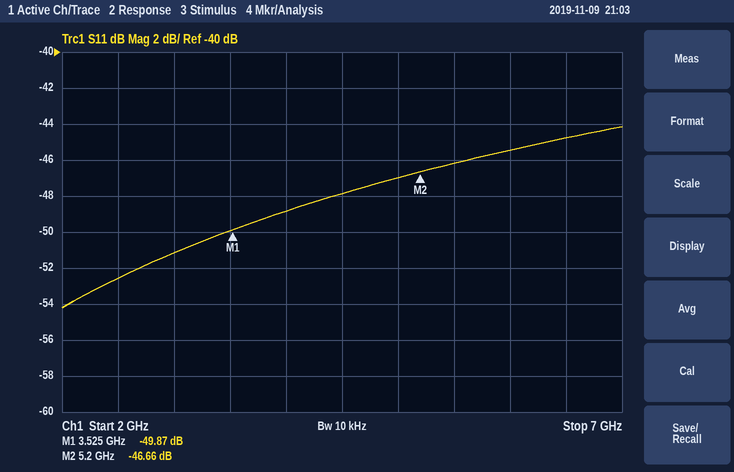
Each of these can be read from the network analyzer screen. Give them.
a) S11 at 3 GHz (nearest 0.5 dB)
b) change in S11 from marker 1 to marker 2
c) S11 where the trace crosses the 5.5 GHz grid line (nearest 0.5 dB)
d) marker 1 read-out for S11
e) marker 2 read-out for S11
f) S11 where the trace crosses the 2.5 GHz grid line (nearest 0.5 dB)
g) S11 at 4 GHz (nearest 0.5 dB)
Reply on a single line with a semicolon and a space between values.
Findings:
-51.0 dB; 3.21 dB; -46.0 dB; -49.87 dB; -46.66 dB; -52.5 dB; -49.0 dB
